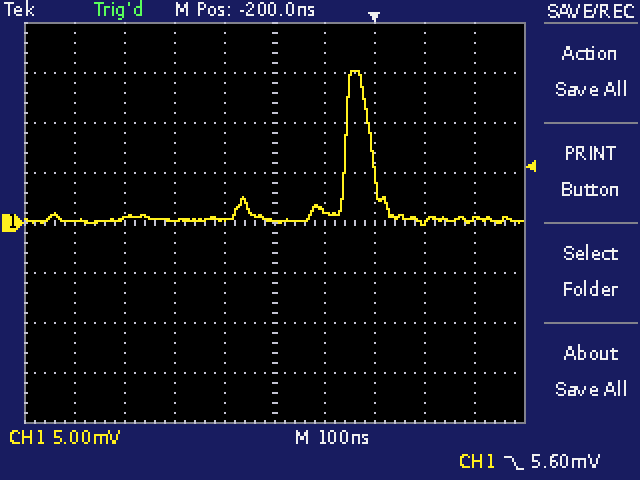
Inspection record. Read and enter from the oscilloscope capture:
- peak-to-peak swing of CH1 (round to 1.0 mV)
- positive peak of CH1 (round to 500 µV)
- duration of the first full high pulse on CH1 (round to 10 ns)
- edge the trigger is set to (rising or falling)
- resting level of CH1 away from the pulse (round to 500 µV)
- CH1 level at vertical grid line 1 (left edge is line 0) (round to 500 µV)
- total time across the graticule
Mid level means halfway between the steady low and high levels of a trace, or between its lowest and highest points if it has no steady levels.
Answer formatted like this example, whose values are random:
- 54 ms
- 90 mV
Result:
- 15.0 mV
- 15.0 mV
- 50 ns
- falling
- 500 µV
- 0.0 mV
- 1 µs
